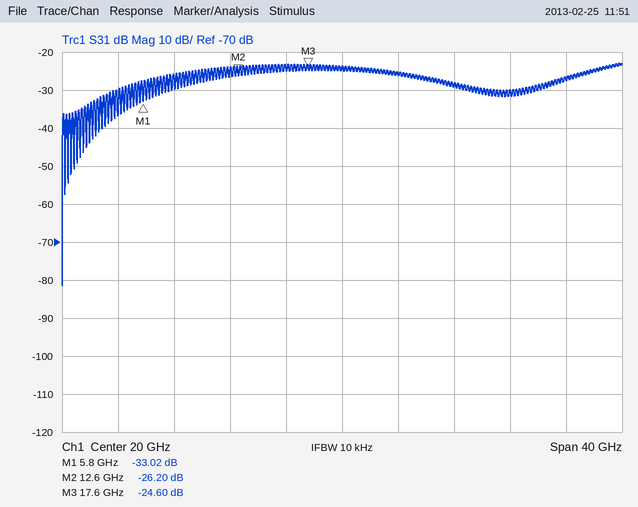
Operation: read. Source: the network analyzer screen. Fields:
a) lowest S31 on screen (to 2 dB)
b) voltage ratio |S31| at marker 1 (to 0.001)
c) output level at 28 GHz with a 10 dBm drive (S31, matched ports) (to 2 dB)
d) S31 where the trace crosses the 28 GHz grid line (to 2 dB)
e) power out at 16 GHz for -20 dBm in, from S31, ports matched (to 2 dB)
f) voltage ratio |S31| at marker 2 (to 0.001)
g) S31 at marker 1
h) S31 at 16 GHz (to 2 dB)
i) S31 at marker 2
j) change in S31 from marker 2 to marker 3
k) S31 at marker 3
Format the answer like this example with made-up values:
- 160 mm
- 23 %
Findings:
- -82 dB
- 0.022
- -18 dBm
- -28 dB
- -44 dBm
- 0.049
- -33.02 dB
- -24 dB
- -26.20 dB
- 1.60 dB
- -24.60 dB
